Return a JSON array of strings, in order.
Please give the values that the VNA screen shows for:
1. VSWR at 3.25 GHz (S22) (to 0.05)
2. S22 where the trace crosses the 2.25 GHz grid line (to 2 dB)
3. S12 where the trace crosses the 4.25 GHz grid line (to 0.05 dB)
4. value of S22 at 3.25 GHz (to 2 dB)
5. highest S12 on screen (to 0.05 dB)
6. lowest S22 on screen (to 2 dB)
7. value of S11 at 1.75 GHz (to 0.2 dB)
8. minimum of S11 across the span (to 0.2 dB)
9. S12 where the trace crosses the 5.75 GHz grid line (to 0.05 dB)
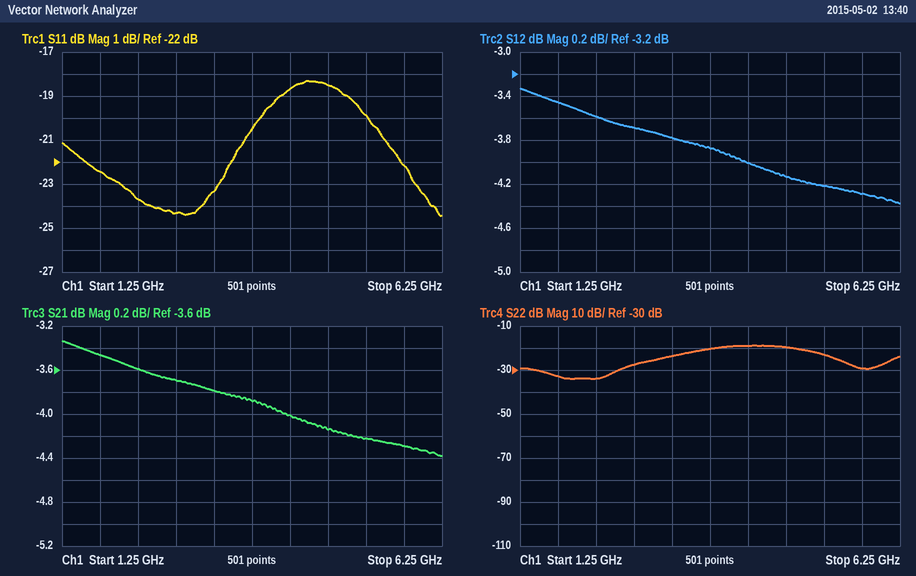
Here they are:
["1.15", "-34 dB", "-4.00 dB", "-24 dB", "-3.35 dB", "-34 dB", "-22.4 dB", "-24.4 dB", "-4.30 dB"]
